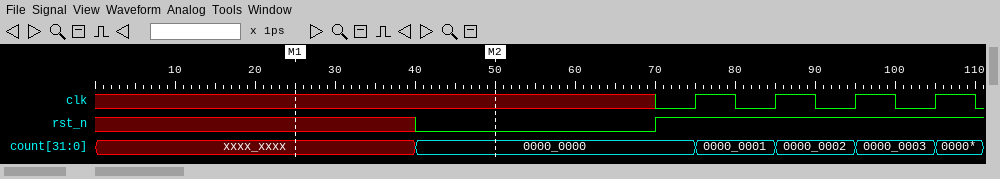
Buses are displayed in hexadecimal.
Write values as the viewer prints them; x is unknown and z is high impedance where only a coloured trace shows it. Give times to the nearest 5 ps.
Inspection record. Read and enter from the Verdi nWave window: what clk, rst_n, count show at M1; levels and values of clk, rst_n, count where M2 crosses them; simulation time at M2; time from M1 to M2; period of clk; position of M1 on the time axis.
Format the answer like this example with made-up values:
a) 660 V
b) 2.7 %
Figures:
a) clk=x, rst_n=x, count=xxxx_xxxx
b) clk=x, rst_n=0, count=0000_0000
c) 50 ps
d) 25 ps
e) 10 ps
f) 25 ps
